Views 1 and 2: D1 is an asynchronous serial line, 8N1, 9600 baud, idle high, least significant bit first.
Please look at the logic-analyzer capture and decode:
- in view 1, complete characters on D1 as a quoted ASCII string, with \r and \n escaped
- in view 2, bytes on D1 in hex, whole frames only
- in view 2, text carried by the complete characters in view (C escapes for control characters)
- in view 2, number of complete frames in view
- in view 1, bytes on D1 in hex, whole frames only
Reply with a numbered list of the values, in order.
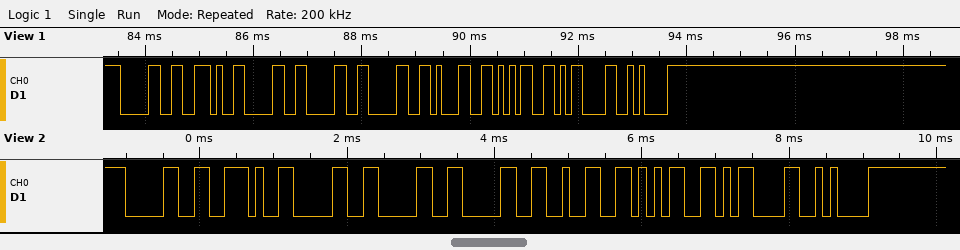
1. "0.00015\r\n"
2. 30 2E 30 30 30 32 35 0D 0A
3. "0.00025\r\n"
4. 9
5. 0x30 0x2E 0x30 0x30 0x30 0x31 0x35 0x0D 0x0A
